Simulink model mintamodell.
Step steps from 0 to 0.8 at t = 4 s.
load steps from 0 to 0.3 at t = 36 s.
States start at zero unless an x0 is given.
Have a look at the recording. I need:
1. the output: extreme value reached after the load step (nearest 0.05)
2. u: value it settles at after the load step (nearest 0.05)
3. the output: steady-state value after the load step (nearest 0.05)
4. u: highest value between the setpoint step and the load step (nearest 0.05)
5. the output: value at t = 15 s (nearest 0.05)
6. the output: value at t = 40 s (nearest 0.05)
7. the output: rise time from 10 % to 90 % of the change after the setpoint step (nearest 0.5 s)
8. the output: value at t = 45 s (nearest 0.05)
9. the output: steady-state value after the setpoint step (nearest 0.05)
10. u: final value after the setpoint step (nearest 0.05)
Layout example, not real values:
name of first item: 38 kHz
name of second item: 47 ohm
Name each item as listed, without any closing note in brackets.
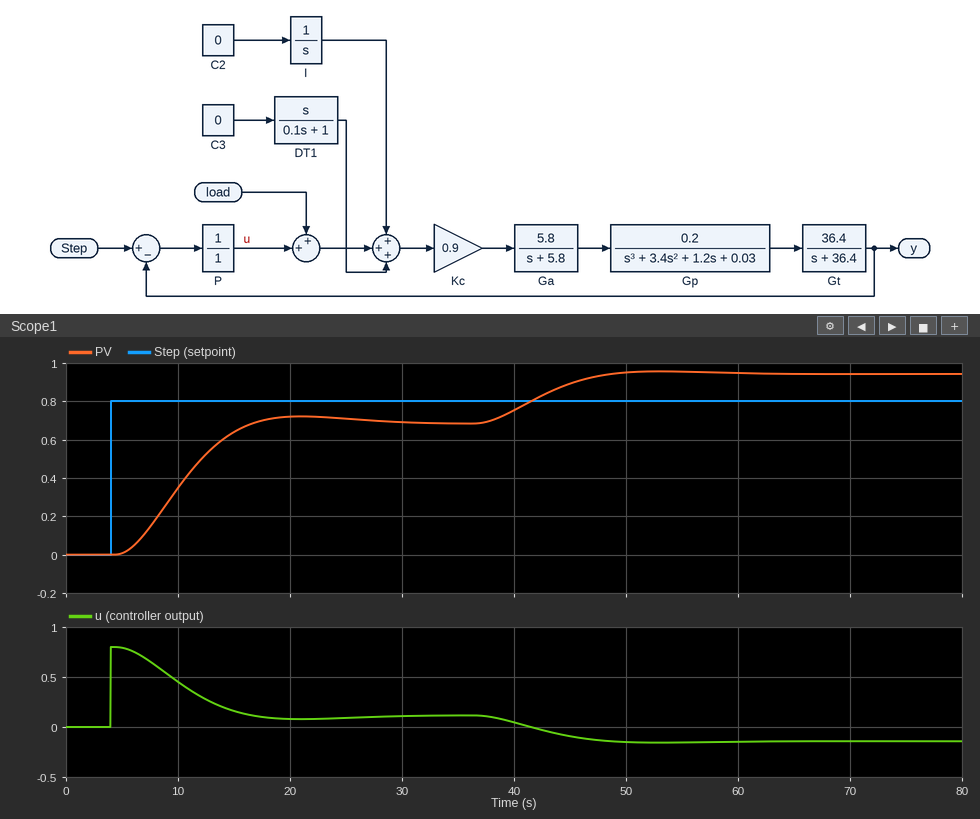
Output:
the output: extreme value reached after the load step: 0.95
u: value it settles at after the load step: -0.15
the output: steady-state value after the load step: 0.95
u: highest value between the setpoint step and the load step: 0.80
the output: value at t = 15 s: 0.65
the output: value at t = 40 s: 0.75
the output: rise time from 10 % to 90 % of the change after the setpoint step: 8.0 s
the output: value at t = 45 s: 0.90
the output: steady-state value after the setpoint step: 0.70
u: final value after the setpoint step: 0.10
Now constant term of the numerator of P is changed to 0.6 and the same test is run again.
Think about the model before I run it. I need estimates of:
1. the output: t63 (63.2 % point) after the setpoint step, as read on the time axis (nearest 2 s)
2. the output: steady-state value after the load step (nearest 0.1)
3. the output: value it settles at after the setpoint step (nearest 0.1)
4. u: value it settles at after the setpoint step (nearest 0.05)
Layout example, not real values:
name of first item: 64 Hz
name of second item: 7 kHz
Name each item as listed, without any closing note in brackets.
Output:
the output: t63 (63.2 % point) after the setpoint step, as read on the time axis: 14 s
the output: steady-state value after the load step: 1.0
the output: value it settles at after the setpoint step: 0.6
u: value it settles at after the setpoint step: 0.10
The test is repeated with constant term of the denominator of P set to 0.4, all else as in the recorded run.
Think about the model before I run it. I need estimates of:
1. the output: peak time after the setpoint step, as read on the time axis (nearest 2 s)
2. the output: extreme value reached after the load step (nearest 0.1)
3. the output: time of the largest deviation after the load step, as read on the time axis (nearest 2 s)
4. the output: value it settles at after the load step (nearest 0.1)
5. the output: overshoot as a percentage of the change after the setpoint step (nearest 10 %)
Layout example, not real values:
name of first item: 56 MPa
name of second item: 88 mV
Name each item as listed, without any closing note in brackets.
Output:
the output: peak time after the setpoint step, as read on the time axis: 14 s
the output: extreme value reached after the load step: 0.9
the output: time of the largest deviation after the load step, as read on the time axis: 46 s
the output: value it settles at after the load step: 0.9
the output: overshoot as a percentage of the change after the setpoint step: 30 %
